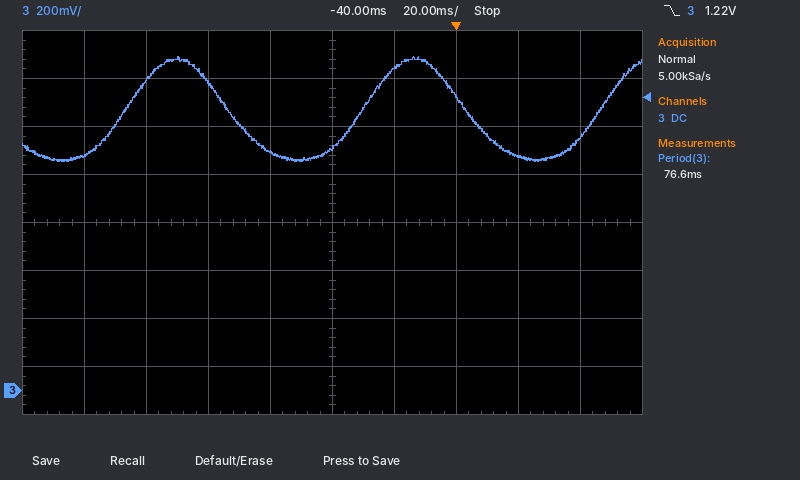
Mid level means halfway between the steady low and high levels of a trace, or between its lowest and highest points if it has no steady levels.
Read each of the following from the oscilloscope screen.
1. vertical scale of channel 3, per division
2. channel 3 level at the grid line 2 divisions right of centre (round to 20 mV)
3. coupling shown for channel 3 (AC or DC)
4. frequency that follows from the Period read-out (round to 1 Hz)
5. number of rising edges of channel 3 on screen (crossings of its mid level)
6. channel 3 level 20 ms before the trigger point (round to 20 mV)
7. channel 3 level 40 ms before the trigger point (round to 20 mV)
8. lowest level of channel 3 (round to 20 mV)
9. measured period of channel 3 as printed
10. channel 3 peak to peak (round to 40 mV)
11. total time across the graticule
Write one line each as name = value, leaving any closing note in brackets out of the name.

vertical scale of channel 3, per division = 200 mV
channel 3 level at the grid line 2 divisions right of centre = 1.22 V
coupling shown for channel 3 = DC
frequency that follows from the Period read-out = 13 Hz
number of rising edges of channel 3 on screen = 3
channel 3 level 20 ms before the trigger point = 1.34 V
channel 3 level 40 ms before the trigger point = 1.00 V
lowest level of channel 3 = 960 mV
measured period of channel 3 as printed = 76.6 ms
channel 3 peak to peak = 440 mV
total time across the graticule = 200 ms
